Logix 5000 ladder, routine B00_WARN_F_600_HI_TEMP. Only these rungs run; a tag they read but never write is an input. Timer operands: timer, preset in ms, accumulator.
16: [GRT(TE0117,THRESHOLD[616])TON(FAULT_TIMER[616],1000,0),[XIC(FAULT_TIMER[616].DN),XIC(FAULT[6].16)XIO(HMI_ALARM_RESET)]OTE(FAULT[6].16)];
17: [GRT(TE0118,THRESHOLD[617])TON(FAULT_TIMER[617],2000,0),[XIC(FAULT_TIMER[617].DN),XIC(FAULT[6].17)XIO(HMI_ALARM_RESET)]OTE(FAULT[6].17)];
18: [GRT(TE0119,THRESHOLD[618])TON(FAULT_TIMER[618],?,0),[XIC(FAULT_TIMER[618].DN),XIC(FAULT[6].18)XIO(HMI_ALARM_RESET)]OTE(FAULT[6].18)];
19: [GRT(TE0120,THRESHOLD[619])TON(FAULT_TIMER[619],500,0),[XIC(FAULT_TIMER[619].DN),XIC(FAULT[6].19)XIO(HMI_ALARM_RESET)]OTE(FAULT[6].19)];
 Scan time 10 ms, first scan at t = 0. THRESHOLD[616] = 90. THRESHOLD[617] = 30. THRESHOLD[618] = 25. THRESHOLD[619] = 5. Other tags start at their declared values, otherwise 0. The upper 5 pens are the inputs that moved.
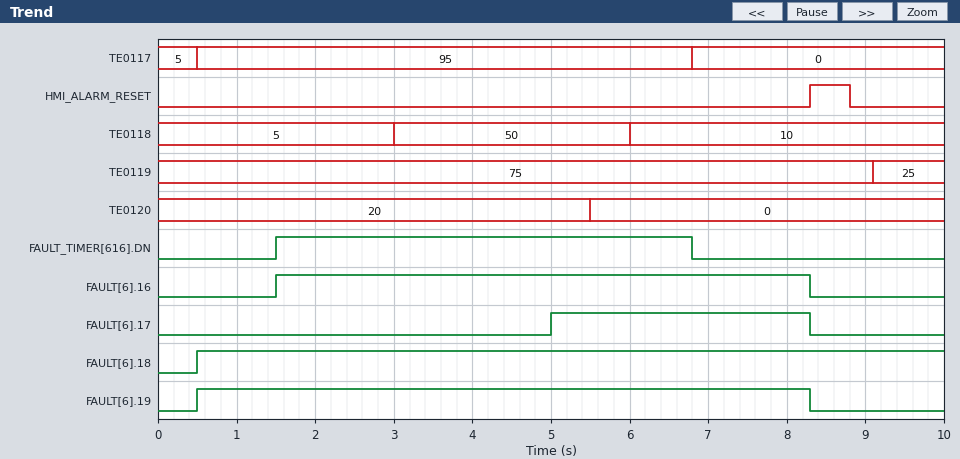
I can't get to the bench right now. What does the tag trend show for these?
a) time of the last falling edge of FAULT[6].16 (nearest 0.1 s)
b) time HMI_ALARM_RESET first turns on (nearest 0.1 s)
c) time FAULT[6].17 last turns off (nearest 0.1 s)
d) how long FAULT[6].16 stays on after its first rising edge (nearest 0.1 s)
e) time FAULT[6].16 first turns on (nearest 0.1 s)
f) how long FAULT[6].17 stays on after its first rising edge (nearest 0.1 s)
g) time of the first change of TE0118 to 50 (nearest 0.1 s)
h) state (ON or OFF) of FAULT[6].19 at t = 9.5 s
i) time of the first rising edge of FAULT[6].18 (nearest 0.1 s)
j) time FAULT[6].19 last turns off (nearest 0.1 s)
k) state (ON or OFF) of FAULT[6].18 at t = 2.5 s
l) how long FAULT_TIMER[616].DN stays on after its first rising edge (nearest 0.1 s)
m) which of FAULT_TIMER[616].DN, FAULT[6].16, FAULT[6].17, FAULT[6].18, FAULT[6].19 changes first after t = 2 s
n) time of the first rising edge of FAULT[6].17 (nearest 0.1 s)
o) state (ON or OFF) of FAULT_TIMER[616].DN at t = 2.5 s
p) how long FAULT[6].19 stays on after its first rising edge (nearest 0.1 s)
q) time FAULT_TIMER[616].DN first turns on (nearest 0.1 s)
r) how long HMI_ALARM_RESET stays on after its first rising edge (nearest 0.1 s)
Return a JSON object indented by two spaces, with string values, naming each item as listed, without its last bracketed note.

{
  "time of the last falling edge of FAULT[6].16": "8.3 s",
  "time HMI_ALARM_RESET first turns on": "8.3 s",
  "time FAULT[6].17 last turns off": "8.3 s",
  "how long FAULT[6].16 stays on after its first rising edge": "6.8 s",
  "time FAULT[6].16 first turns on": "1.5 s",
  "how long FAULT[6].17 stays on after its first rising edge": "3.3 s",
  "time of the first change of TE0118 to 50": "3.0 s",
  "state (ON or OFF) of FAULT[6].19 at t = 9.5 s": "OFF",
  "time of the first rising edge of FAULT[6].18": "0.5 s",
  "time FAULT[6].19 last turns off": "8.3 s",
  "state (ON or OFF) of FAULT[6].18 at t = 2.5 s": "ON",
  "how long FAULT_TIMER[616].DN stays on after its first rising edge": "5.3 s",
  "which of FAULT_TIMER[616].DN, FAULT[6].16, FAULT[6].17, FAULT[6].18, FAULT[6].19 changes first after t = 2 s": "FAULT[6].17",
  "time of the first rising edge of FAULT[6].17": "5.0 s",
  "state (ON or OFF) of FAULT_TIMER[616].DN at t = 2.5 s": "ON",
  "how long FAULT[6].19 stays on after its first rising edge": "7.8 s",
  "time FAULT_TIMER[616].DN first turns on": "1.5 s",
  "how long HMI_ALARM_RESET stays on after its first rising edge": "0.5 s"
}
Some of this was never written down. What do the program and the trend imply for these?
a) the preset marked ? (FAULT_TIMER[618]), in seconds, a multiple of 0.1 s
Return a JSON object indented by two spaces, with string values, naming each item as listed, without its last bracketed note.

{
  "the preset marked ? (FAULT_TIMER[618]), in seconds, a multiple of 0.1 s": "0.5 s"
}
